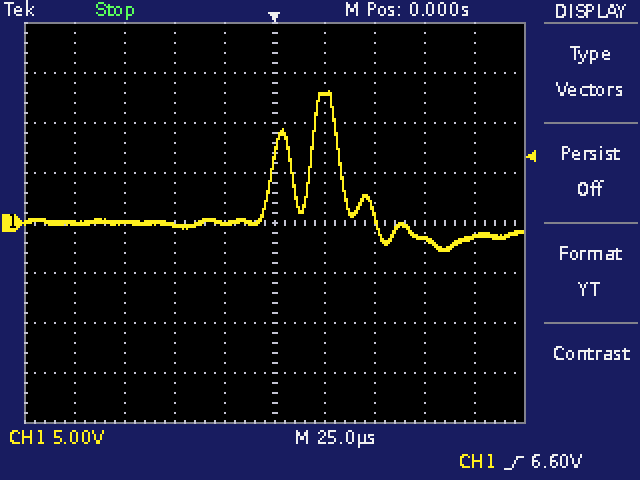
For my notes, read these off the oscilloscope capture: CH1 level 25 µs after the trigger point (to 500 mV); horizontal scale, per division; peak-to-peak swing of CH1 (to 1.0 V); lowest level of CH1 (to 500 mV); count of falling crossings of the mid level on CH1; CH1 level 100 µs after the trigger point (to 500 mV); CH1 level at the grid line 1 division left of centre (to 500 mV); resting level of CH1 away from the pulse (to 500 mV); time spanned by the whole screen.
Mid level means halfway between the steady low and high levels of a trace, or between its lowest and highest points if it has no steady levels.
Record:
13.0 V
25 µs
16.0 V
-3.0 V
2
-1.5 V
0.0 V
0.0 V
250 µs
